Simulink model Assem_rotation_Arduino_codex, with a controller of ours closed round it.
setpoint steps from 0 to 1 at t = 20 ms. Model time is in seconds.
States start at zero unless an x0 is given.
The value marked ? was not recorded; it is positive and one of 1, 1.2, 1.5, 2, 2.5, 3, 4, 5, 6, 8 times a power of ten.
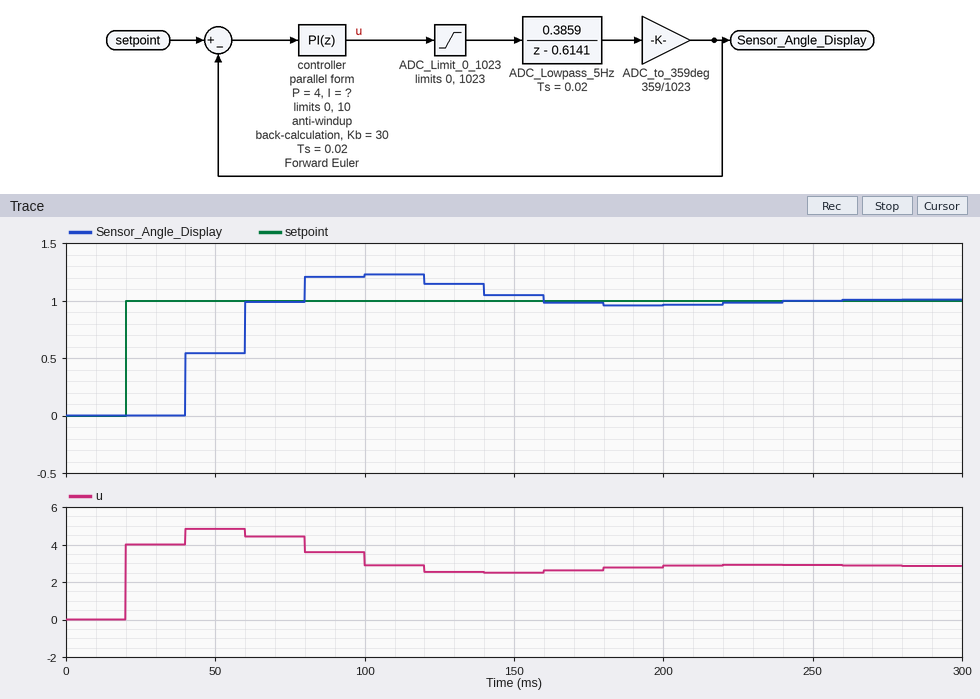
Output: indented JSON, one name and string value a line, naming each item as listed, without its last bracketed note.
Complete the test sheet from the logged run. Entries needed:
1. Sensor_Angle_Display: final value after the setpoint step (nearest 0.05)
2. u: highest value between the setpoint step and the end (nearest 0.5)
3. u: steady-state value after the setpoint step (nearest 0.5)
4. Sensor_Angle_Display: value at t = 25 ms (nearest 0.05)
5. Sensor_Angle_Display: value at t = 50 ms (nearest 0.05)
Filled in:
{
  "Sensor_Angle_Display: final value after the setpoint step": "1.00",
  "u: highest value between the setpoint step and the end": "5.0",
  "u: steady-state value after the setpoint step": "3.0",
  "Sensor_Angle_Display: value at t = 25 ms": "0.00",
  "Sensor_Angle_Display: value at t = 50 ms": "0.55"
}
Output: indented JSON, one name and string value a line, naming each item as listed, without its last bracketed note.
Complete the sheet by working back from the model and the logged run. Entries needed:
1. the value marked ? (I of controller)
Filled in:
{
  "the value marked ?": "150"
}
